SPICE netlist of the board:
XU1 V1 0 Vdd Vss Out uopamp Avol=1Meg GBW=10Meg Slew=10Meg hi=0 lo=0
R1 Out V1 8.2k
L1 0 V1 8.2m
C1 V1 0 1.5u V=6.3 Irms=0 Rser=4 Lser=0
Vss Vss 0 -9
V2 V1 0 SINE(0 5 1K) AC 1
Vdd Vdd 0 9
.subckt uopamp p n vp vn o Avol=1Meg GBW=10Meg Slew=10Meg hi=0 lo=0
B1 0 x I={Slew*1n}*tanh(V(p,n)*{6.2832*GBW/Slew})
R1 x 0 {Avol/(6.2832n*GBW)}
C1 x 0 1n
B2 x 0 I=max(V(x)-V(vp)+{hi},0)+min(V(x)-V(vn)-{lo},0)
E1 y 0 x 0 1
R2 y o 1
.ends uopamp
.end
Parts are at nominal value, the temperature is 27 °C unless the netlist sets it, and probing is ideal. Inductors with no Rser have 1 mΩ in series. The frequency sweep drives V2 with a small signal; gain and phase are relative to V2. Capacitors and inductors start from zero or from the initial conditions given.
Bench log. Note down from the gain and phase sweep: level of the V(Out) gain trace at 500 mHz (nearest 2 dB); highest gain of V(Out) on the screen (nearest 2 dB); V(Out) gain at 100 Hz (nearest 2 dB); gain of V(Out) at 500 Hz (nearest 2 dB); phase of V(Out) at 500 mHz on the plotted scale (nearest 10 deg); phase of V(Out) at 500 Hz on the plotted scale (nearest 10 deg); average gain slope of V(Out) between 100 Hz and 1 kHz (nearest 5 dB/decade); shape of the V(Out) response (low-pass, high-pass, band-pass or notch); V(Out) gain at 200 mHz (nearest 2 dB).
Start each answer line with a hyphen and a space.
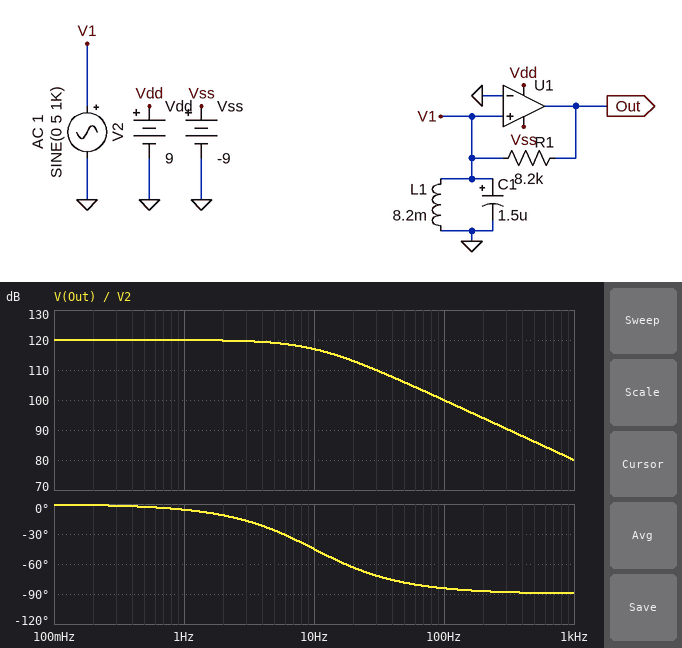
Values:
- 120 dB
- 120 dB
- 100 dB
- 86 dB
- 0 deg
- -90 deg
- -20 dB/decade
- low-pass
- 120 dB
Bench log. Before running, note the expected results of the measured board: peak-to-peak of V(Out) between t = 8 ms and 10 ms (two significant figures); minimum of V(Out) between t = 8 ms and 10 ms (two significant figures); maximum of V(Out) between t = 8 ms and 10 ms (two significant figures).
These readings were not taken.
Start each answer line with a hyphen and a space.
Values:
- 18 V
- -9.0 V
- 9.0 V
